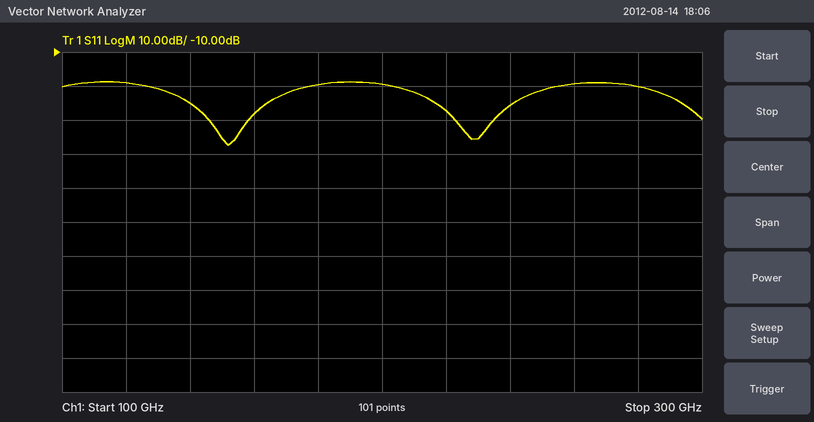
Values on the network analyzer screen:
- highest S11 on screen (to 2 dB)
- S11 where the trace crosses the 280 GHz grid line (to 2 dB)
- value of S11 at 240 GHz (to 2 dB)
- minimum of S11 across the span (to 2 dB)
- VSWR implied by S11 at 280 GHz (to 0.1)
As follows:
-18 dB
-20 dB
-26 dB
-38 dB
1.2
